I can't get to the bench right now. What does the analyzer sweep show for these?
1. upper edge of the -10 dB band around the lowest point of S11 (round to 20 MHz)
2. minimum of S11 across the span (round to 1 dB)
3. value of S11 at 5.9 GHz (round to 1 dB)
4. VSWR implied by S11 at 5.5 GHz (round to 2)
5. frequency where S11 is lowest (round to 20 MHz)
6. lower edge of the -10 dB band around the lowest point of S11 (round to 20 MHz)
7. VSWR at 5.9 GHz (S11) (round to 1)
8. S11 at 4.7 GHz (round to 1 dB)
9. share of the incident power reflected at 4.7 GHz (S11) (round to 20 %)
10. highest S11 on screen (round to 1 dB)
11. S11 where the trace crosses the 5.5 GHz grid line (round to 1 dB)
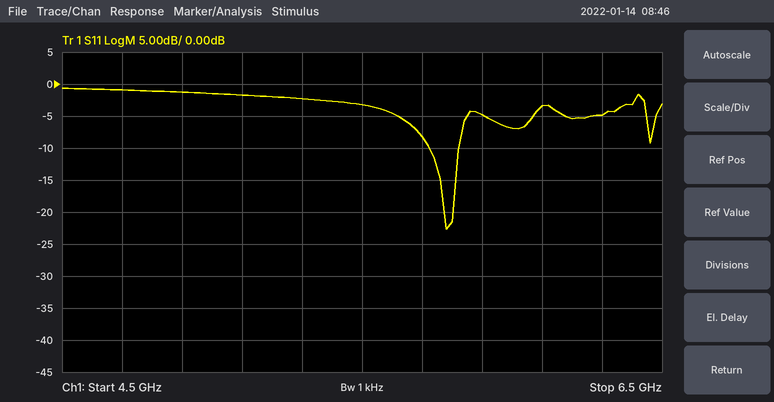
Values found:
5.82 GHz
-23 dB
-5 dB
6
5.78 GHz
5.72 GHz
4
-1 dB
80 %
-1 dB
-3 dB
